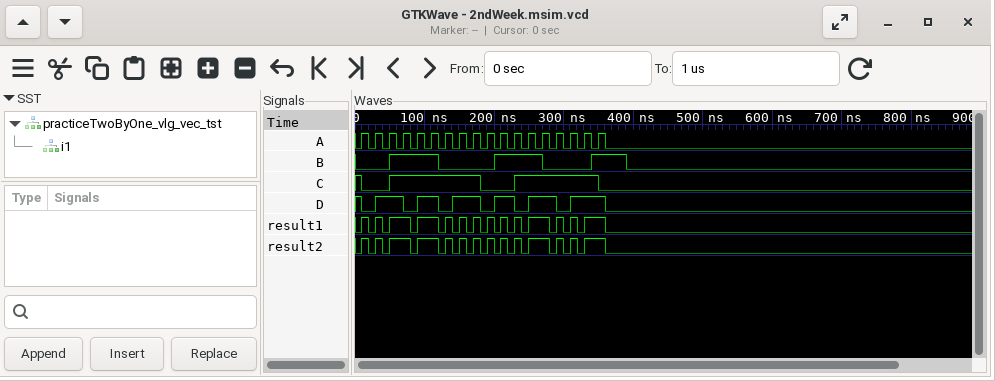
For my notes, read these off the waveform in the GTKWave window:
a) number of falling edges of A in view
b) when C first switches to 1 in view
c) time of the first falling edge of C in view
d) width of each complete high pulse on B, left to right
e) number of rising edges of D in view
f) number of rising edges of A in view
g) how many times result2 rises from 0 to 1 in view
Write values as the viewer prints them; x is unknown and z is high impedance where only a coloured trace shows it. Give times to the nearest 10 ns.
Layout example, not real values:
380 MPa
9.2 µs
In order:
18
50 ns
10 ns
70 ns, 70 ns, 50 ns
6
18
14
